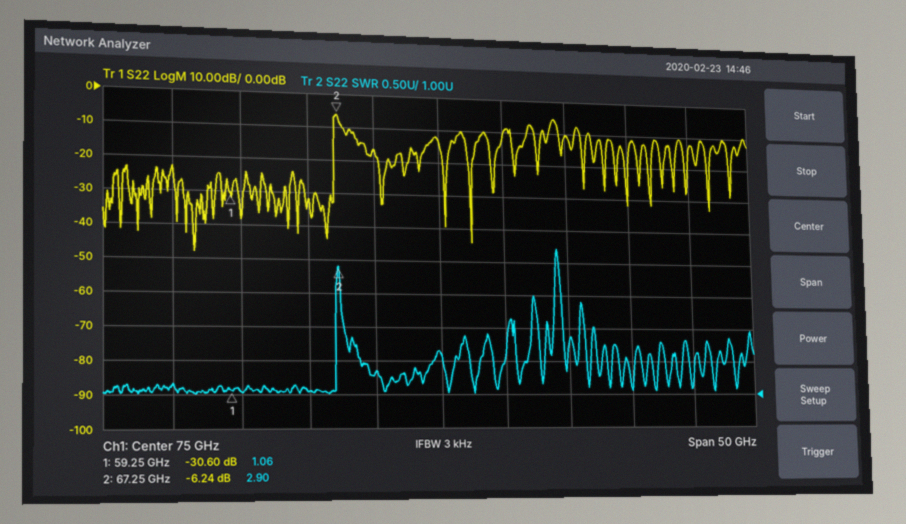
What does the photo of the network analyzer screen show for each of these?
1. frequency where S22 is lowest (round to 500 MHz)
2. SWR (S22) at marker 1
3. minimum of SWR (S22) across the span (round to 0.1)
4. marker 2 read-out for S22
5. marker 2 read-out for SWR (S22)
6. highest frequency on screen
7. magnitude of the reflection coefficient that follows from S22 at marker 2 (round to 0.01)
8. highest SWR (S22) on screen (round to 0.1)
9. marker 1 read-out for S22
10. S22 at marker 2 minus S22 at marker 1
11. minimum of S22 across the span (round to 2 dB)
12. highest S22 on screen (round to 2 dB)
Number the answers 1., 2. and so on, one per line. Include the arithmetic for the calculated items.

1. 56.5 GHz
2. 1.06
3. 1.0
4. -6.24 dB
5. 2.90
6. 100 GHz
7. 10^(-6.24/20) ≈ 0.49
8. 3.2
9. -30.60 dB
10. -6.24 − (-30.6) = 24.36 dB
11. -48 dB
12. -6 dB
